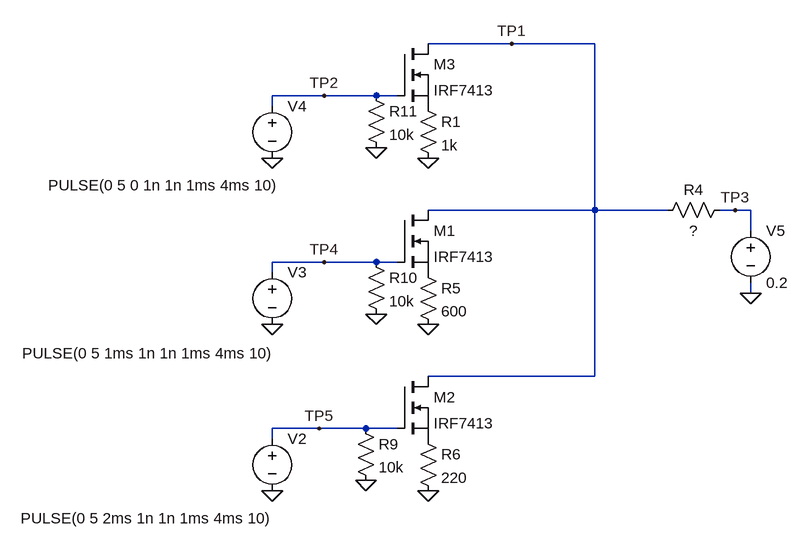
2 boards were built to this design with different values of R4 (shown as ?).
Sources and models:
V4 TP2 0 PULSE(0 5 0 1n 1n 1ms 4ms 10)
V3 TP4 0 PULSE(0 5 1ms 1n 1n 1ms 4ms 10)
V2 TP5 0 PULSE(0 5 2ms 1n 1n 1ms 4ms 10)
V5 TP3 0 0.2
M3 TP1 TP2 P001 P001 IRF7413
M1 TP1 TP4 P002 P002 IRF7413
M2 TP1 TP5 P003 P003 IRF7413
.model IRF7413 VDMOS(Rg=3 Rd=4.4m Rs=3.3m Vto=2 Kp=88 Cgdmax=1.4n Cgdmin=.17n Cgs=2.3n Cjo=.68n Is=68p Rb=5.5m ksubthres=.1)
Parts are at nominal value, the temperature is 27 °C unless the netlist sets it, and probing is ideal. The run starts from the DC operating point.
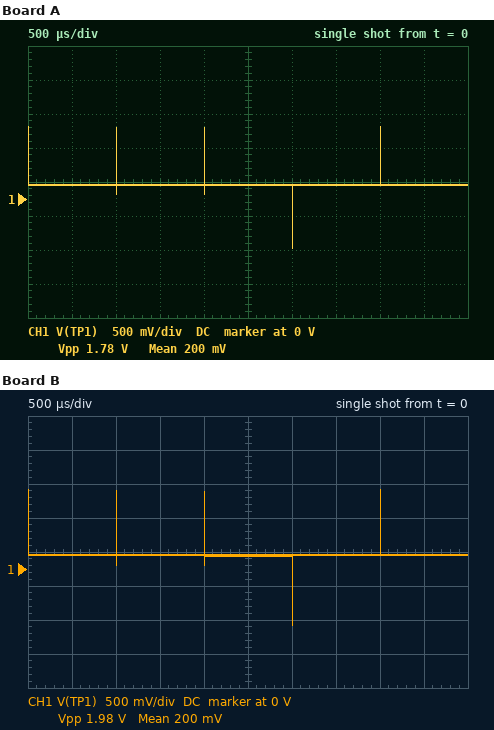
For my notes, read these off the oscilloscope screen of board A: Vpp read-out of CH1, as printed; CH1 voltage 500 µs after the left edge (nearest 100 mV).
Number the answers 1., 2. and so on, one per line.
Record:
1. 1.78 V
2. 200 mV
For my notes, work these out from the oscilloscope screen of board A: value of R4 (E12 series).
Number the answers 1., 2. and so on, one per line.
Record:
1. 1.2 Ω
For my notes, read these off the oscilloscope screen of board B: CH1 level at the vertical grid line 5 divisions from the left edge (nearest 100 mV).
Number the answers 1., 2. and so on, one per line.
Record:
1. 200 mV
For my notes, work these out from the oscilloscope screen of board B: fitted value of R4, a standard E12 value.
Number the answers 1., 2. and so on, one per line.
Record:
1. 1.5 Ω
